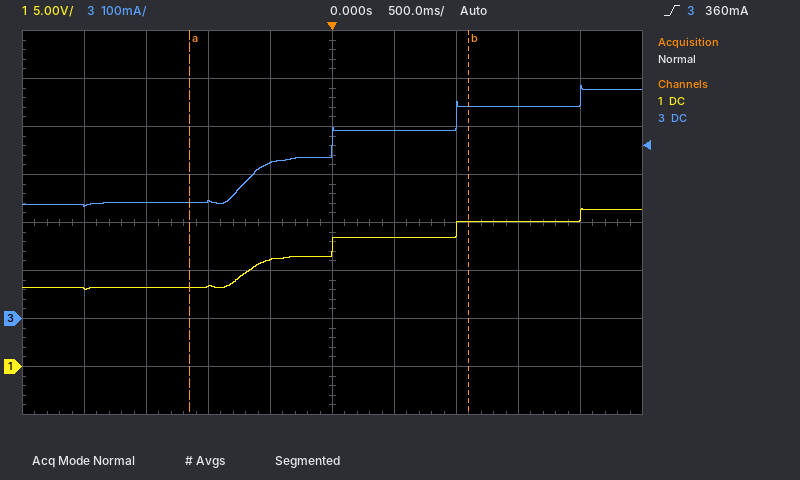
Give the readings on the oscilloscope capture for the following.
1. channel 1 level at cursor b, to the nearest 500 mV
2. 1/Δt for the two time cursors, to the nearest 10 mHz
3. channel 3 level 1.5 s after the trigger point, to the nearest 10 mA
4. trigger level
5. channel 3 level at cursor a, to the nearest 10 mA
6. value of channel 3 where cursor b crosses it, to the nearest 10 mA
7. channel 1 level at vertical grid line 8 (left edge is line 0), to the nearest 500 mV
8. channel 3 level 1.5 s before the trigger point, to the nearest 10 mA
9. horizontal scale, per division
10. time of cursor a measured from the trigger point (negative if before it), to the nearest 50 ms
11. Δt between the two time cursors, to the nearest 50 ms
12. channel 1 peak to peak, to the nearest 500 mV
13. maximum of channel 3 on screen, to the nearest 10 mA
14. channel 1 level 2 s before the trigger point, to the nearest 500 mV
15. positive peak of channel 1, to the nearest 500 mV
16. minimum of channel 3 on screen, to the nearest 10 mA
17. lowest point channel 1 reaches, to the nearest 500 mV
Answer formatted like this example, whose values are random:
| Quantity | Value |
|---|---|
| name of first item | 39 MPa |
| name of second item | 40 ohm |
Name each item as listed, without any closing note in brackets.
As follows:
| Quantity | Value |
|---|---|
| channel 1 level at cursor b, to the nearest 500 mV | 15.0 V |
| 1/Δt for the two time cursors, to the nearest 10 mHz | 440 mHz |
| channel 3 level 1.5 s after the trigger point, to the nearest 10 mA | 440 mA |
| trigger level | 360 mA |
| channel 3 level at cursor a, to the nearest 10 mA | 240 mA |
| value of channel 3 where cursor b crosses it, to the nearest 10 mA | 440 mA |
| channel 1 level at vertical grid line 8 (left edge is line 0), to the nearest 500 mV | 15.0 V |
| channel 3 level 1.5 s before the trigger point, to the nearest 10 mA | 240 mA |
| horizontal scale, per division | 500 ms |
| time of cursor a measured from the trigger point (negative if before it), to the nearest 50 ms | -1.15 s |
| Δt between the two time cursors, to the nearest 50 ms | 2.25 s |
| channel 1 peak to peak, to the nearest 500 mV | 8.5 V |
| maximum of channel 3 on screen, to the nearest 10 mA | 490 mA |
| channel 1 level 2 s before the trigger point, to the nearest 500 mV | 8.0 V |
| positive peak of channel 1, to the nearest 500 mV | 16.5 V |
| minimum of channel 3 on screen, to the nearest 10 mA | 230 mA |
| lowest point channel 1 reaches, to the nearest 500 mV | 8.0 V |
